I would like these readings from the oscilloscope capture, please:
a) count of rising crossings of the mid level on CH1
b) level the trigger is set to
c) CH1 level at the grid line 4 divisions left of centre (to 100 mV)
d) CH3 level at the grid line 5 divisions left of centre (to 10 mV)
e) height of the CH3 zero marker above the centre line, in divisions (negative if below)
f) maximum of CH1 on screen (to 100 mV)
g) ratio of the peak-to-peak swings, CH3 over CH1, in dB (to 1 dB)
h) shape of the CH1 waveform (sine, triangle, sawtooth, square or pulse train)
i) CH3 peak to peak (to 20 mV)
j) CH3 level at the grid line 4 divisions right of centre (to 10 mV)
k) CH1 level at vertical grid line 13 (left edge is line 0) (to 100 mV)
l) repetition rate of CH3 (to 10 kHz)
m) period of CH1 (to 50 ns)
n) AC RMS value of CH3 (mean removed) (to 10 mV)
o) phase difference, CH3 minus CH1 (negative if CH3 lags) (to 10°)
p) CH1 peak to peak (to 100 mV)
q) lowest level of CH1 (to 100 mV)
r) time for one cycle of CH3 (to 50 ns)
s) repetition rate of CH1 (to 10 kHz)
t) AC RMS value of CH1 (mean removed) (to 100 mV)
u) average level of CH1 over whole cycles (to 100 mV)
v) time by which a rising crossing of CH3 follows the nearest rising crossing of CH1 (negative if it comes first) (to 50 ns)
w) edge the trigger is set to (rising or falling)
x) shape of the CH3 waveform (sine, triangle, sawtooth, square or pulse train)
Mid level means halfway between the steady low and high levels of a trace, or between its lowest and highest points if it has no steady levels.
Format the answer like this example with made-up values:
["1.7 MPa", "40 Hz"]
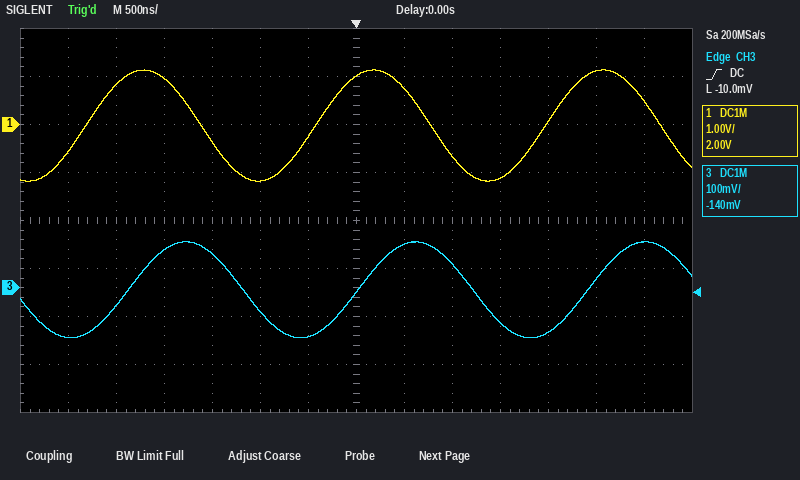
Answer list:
["3", "-10.0 mV", "1.0 V", "-40 mV", "-1.4 div", "1.1 V", "-21 dB", "sine", "200 mV", "-90 mV", "500 mV", "420 kHz", "2.40 µs", "70 mV", "-70°", "2.3 V", "-1.2 V", "2.40 µs", "420 kHz", "800 mV", "0.0 V", "+450 ns", "rising", "sine"]
